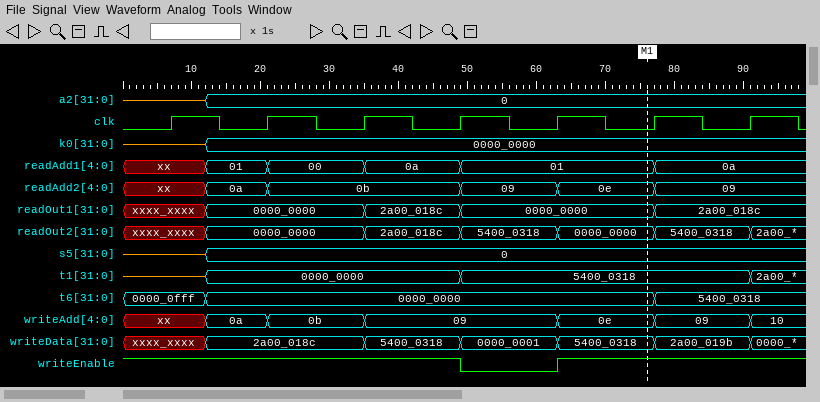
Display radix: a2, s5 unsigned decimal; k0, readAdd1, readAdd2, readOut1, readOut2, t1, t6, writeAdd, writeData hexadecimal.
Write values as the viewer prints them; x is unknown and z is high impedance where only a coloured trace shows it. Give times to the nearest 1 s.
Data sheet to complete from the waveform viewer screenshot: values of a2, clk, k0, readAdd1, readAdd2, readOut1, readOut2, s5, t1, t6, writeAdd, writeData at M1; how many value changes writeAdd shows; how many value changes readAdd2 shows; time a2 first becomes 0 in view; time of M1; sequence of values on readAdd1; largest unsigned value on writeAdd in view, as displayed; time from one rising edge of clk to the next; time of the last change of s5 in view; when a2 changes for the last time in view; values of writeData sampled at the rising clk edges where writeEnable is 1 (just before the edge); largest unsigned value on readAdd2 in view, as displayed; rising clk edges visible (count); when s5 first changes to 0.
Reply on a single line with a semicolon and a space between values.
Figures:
a2=0, clk=0, k0=0000_0000, readAdd1=01, readAdd2=0e, readOut1=0000_0000, readOut2=0000_0000, s5=0, t1=5400_0318, t6=0000_0000, writeAdd=0e, writeData=5400_0318; 6; 5; 12 s; 76 s; xx, 01, 00, 0a, 01, 0a; 10; 14 s; 12 s; 12 s; xxxx_xxxx, 2a00_018c, 2a00_018c, 5400_0318, 5400_0318, 2a00_019b; 0e; 7; 12 s
